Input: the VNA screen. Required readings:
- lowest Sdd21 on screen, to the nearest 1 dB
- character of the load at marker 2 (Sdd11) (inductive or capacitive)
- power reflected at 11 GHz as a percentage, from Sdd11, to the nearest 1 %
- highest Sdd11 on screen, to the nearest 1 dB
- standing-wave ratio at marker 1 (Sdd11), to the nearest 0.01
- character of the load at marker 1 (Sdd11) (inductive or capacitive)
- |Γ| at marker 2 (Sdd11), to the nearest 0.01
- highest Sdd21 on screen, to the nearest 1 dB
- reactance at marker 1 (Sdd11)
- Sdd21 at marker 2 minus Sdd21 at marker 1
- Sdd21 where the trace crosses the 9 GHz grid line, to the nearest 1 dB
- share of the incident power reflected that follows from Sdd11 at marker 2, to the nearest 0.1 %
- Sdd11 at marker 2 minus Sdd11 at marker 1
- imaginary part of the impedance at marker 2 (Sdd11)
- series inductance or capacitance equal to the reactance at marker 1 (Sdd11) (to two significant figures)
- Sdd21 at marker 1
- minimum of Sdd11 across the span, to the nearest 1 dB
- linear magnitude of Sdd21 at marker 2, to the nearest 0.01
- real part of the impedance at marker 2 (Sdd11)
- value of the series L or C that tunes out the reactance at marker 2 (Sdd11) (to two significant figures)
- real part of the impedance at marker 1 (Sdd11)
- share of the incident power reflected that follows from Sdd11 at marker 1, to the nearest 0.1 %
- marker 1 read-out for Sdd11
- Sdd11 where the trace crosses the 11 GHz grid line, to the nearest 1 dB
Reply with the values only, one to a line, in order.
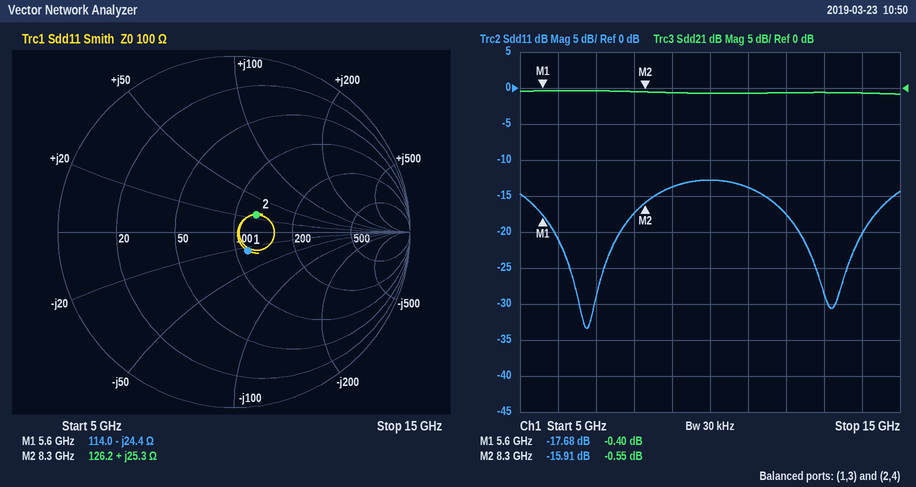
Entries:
-1 dB
inductive
4 %
-13 dB
1.30
capacitive
0.16
0 dB
-24.4 Ω
-0.15 dB
-1 dB
2.6 %
1.77 dB
+25.3 Ω
1.2 pF
-0.40 dB
-33 dB
0.94
126.2 Ω
760 fF
114.0 Ω
1.7 %
-17.68 dB
-14 dB
